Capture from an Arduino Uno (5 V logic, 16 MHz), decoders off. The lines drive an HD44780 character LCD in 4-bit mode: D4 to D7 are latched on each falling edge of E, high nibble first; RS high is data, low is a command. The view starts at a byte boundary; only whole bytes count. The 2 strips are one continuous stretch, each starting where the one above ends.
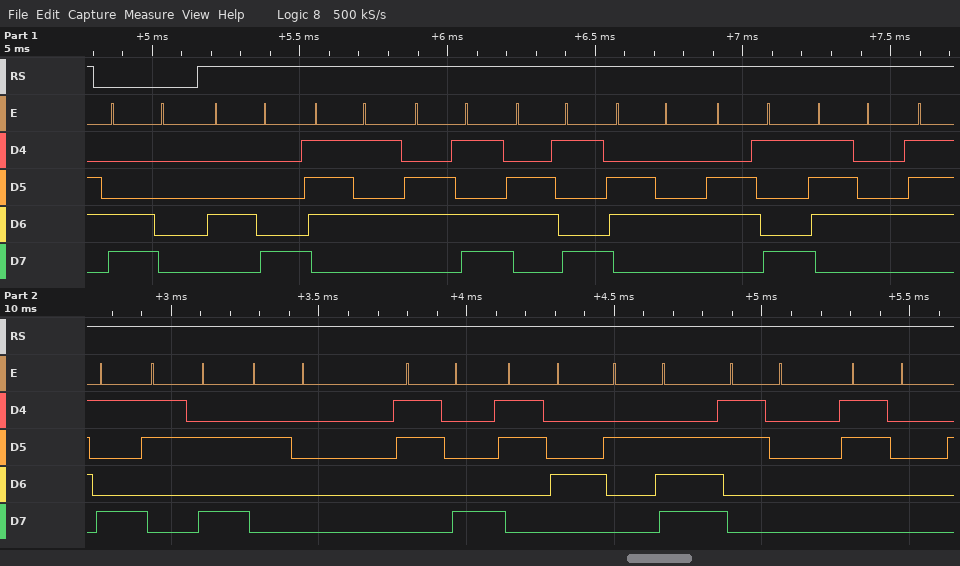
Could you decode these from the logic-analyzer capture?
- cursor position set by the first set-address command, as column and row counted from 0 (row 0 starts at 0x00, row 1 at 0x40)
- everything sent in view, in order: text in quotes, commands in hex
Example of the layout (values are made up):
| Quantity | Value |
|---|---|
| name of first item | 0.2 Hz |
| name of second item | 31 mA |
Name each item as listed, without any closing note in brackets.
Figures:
| Quantity | Value |
|---|---|
| cursor position set by the first set-address command, as column and row counted from 0 | column 0, row 1 |
| everything sent in view, in order: text in quotes, commands in hex | 0xC0 "Humidity: 84.00" |
